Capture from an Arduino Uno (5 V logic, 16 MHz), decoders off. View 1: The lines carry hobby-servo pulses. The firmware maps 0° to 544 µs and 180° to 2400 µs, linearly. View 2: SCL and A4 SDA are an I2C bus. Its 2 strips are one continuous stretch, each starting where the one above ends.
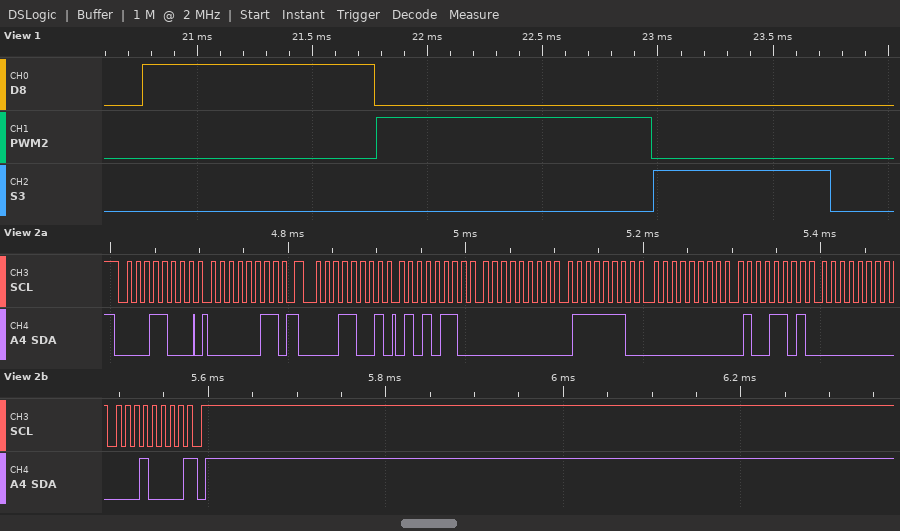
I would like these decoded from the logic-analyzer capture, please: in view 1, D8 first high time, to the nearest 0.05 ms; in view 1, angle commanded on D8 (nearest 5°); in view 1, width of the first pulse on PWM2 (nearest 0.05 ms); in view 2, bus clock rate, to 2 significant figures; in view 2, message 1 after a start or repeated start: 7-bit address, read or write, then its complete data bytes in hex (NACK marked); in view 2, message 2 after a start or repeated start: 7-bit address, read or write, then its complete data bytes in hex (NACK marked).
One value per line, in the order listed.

1.00 ms
45°
1.20 ms
100 kHz
0x0C write: 03
0x0C read: 56 00 7E 00 4D 00 10 NACK
